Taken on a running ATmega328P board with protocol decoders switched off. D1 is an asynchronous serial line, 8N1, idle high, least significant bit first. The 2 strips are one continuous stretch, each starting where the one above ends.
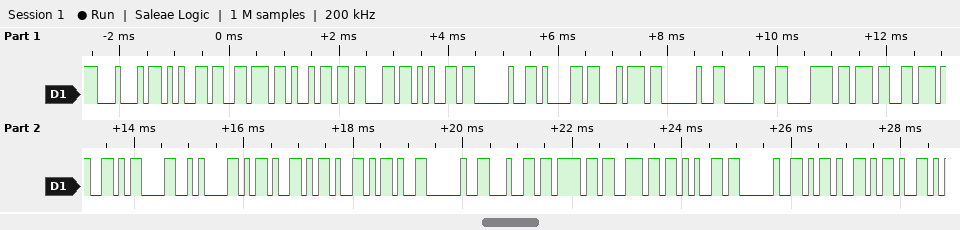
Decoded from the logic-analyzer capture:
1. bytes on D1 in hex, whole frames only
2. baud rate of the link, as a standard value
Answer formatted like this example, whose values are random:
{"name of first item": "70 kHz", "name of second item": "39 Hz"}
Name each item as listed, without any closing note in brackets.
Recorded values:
{"bytes on D1 in hex, whole frames only": "44 65 76 69 63 65 20 61 74 20 30 78 37 37 0D 0A 2D 2D 2D 20 64 6F 6E 65 20 2D 2D", "baud rate of the link, as a standard value": "9600 baud"}
